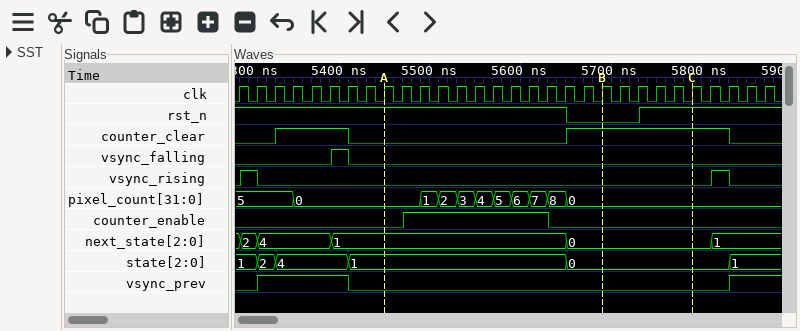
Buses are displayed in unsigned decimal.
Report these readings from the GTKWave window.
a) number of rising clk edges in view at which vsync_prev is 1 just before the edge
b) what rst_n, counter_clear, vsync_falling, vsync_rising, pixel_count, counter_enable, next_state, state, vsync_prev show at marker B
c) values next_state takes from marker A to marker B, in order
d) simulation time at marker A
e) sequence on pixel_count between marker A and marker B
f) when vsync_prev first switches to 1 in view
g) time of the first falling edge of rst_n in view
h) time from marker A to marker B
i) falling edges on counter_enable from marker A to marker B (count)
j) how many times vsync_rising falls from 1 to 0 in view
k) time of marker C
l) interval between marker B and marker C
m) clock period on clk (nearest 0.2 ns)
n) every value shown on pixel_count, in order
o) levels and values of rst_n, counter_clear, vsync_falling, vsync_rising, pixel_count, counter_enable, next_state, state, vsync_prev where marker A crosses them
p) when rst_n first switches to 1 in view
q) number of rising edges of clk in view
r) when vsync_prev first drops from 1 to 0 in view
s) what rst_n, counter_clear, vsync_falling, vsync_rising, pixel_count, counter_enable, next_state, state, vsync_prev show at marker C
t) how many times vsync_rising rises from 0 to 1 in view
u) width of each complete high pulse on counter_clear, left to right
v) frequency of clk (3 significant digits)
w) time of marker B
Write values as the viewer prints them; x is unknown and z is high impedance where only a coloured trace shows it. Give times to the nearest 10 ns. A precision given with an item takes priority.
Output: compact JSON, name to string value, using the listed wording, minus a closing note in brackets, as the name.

{"number of rising clk edges in view at which vsync_prev is 1 just before the edge": "7", "what rst_n, counter_clear, vsync_falling, vsync_rising, pixel_count, counter_enable, next_state, state, vsync_prev show at marker B": "rst_n=0, counter_clear=1, vsync_falling=0, vsync_rising=0, pixel_count=0, counter_enable=0, next_state=0, state=0, vsync_prev=0", "values next_state takes from marker A to marker B, in order": "1, 0", "simulation time at marker A": "5450 ns", "sequence on pixel_count between marker A and marker B": "0, 1, 2, 3, 4, 5, 6, 7, 8, 0", "when vsync_prev first switches to 1 in view": "5310 ns", "time of the first falling edge of rst_n in view": "5650 ns", "time from marker A to marker B": "240 ns", "falling edges on counter_enable from marker A to marker B": "1", "how many times vsync_rising falls from 1 to 0 in view": "2", "time of marker C": "5790 ns", "interval between marker B and marker C": "100 ns", "clock period on clk": "20 ns", "every value shown on pixel_count, in order": "5, 0, 1, 2, 3, 4, 5, 6, 7, 8, 0", "levels and values of rst_n, counter_clear, vsync_falling, vsync_rising, pixel_count, counter_enable, next_state, state, vsync_prev where marker A crosses them": "rst_n=1, counter_clear=0, vsync_falling=0, vsync_rising=0, pixel_count=0, counter_enable=0, next_state=1, state=1, vsync_prev=0", "when rst_n first switches to 1 in view": "5730 ns", "number of rising edges of clk in view": "30", "when vsync_prev first drops from 1 to 0 in view": "5410 ns", "what rst_n, counter_clear, vsync_falling, vsync_rising, pixel_count, counter_enable, next_state, state, vsync_prev show at marker C": "rst_n=1, counter_clear=1, vsync_falling=0, vsync_rising=0, pixel_count=0, counter_enable=0, next_state=0, state=0, vsync_prev=0", "how many times vsync_rising rises from 0 to 1 in view": "2", "width of each complete high pulse on counter_clear, left to right": "80 ns, 180 ns", "frequency of clk": "50.0 MHz", "time of marker B": "5690 ns"}
